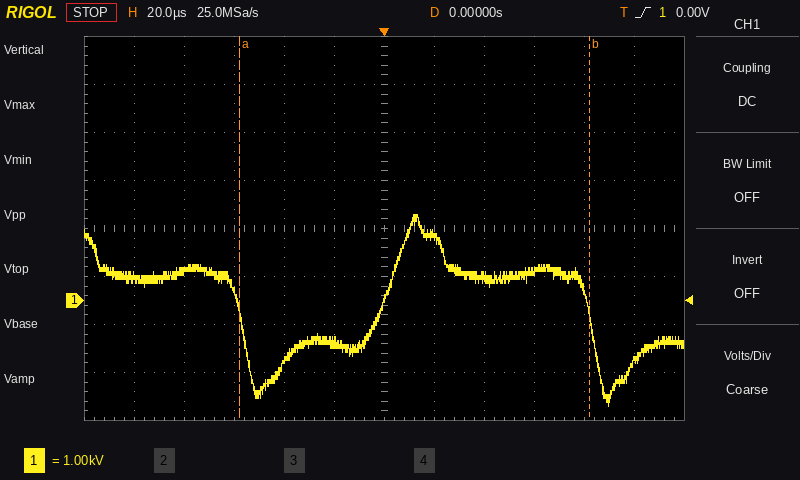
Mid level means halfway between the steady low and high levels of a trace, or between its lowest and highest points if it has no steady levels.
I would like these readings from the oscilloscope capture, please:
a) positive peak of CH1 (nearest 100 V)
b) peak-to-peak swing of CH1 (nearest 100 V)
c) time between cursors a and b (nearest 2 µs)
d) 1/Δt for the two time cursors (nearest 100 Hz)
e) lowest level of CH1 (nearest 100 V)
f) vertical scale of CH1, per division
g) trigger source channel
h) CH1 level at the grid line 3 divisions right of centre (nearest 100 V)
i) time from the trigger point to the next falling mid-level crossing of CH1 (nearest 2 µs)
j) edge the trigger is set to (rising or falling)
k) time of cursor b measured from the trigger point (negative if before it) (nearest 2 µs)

1.8 kV
4.0 kV
140 µs
7.1 kHz
-2.2 kV
1 kV
CH1
600 V
82 µs
rising
+82 µs
